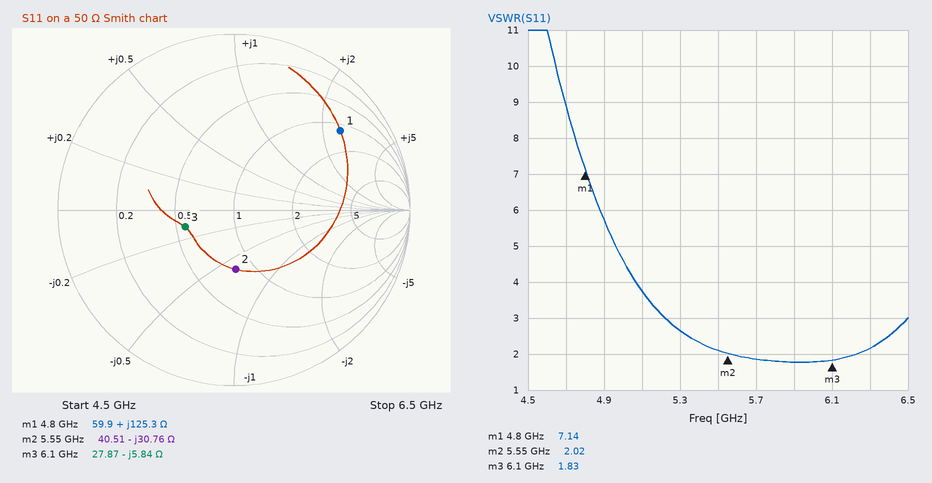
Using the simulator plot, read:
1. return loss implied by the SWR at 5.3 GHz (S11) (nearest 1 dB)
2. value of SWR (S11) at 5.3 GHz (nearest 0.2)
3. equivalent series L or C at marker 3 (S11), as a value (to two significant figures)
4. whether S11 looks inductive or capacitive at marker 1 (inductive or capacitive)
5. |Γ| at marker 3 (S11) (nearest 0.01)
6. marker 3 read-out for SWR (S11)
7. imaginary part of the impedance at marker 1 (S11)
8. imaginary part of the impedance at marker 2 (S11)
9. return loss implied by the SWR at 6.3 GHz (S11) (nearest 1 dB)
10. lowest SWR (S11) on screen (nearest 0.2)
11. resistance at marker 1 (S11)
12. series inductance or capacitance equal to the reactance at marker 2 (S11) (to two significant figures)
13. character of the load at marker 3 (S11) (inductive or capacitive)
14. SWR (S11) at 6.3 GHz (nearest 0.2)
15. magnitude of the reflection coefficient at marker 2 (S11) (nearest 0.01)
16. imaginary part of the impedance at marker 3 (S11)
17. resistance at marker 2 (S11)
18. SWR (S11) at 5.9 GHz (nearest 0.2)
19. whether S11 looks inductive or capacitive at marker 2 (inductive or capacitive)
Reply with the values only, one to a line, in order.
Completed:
7 dB
2.6
4.5 pF
inductive
0.29
1.83
+125.3 Ω
-30.76 Ω
9 dB
1.8
59.9 Ω
930 fF
capacitive
2.2
0.34
-5.84 Ω
40.51 Ω
1.8
capacitive
